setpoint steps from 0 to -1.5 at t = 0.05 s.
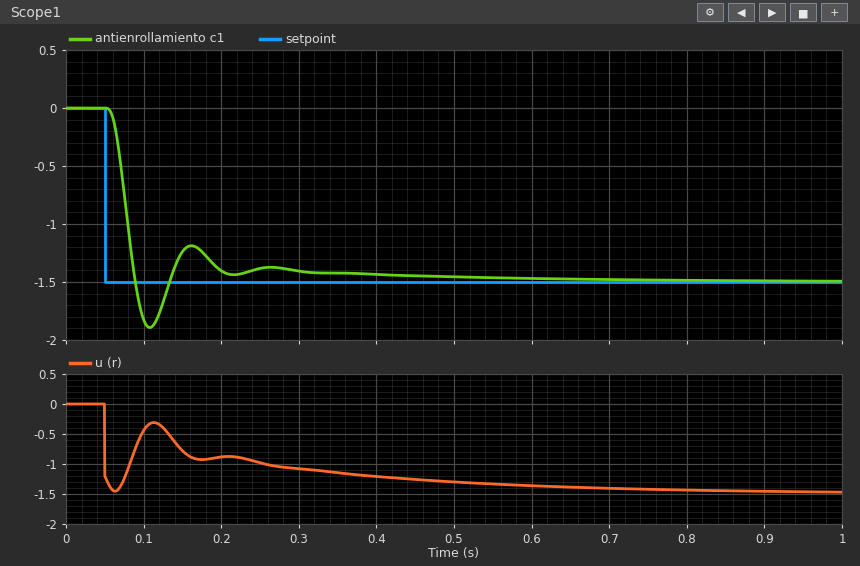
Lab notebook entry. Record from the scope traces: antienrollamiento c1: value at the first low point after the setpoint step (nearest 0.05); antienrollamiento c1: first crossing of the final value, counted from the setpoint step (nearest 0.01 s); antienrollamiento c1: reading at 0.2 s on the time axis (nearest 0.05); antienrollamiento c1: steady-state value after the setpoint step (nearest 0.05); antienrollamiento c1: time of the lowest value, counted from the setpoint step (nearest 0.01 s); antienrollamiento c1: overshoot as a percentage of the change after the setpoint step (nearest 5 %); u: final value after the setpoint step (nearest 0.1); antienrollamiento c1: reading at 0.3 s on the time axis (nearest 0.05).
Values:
-1.90
0.04 s
-1.40
-1.50
0.06 s
25 %
-1.5
-1.40
